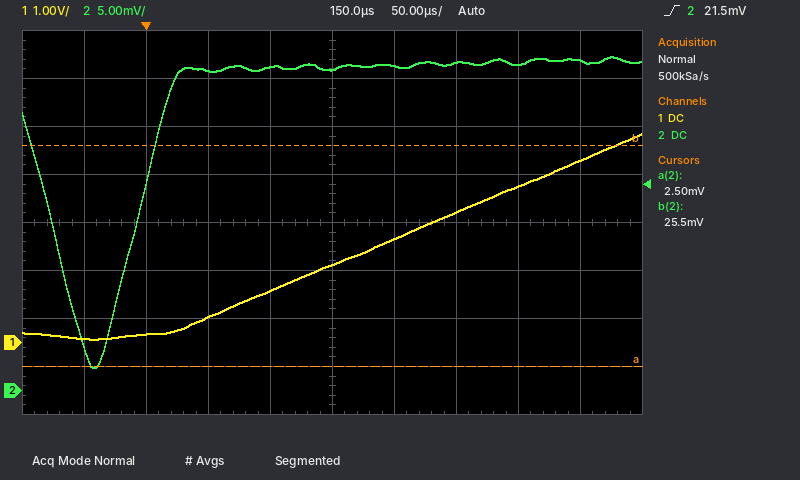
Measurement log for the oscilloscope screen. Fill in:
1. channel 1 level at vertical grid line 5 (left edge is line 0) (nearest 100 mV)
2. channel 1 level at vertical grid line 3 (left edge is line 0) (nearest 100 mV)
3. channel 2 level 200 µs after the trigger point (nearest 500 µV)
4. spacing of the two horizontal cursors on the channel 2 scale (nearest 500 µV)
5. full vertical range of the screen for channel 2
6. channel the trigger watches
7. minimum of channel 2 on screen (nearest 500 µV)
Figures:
1.6 V
500 mV
34.0 mV
23.0 mV
40 mV
channel 2
2.5 mV
